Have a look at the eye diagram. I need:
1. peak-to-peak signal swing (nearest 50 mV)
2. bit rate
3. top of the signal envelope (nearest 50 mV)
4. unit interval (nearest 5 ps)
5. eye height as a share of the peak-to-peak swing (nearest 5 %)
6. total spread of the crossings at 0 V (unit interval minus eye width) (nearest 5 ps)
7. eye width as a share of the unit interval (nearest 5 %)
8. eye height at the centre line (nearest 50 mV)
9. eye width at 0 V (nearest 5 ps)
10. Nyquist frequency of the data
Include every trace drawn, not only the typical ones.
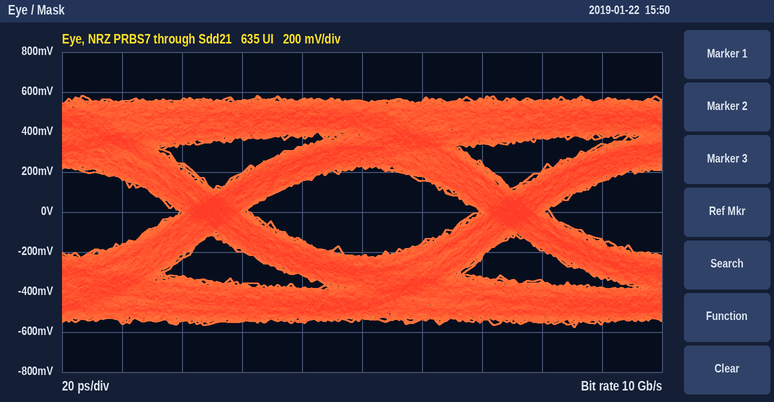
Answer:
1.15 V
10 Gb/s
600 mV
100 ps
40 %
25 ps
75 %
450 mV
75 ps
5 GHz
